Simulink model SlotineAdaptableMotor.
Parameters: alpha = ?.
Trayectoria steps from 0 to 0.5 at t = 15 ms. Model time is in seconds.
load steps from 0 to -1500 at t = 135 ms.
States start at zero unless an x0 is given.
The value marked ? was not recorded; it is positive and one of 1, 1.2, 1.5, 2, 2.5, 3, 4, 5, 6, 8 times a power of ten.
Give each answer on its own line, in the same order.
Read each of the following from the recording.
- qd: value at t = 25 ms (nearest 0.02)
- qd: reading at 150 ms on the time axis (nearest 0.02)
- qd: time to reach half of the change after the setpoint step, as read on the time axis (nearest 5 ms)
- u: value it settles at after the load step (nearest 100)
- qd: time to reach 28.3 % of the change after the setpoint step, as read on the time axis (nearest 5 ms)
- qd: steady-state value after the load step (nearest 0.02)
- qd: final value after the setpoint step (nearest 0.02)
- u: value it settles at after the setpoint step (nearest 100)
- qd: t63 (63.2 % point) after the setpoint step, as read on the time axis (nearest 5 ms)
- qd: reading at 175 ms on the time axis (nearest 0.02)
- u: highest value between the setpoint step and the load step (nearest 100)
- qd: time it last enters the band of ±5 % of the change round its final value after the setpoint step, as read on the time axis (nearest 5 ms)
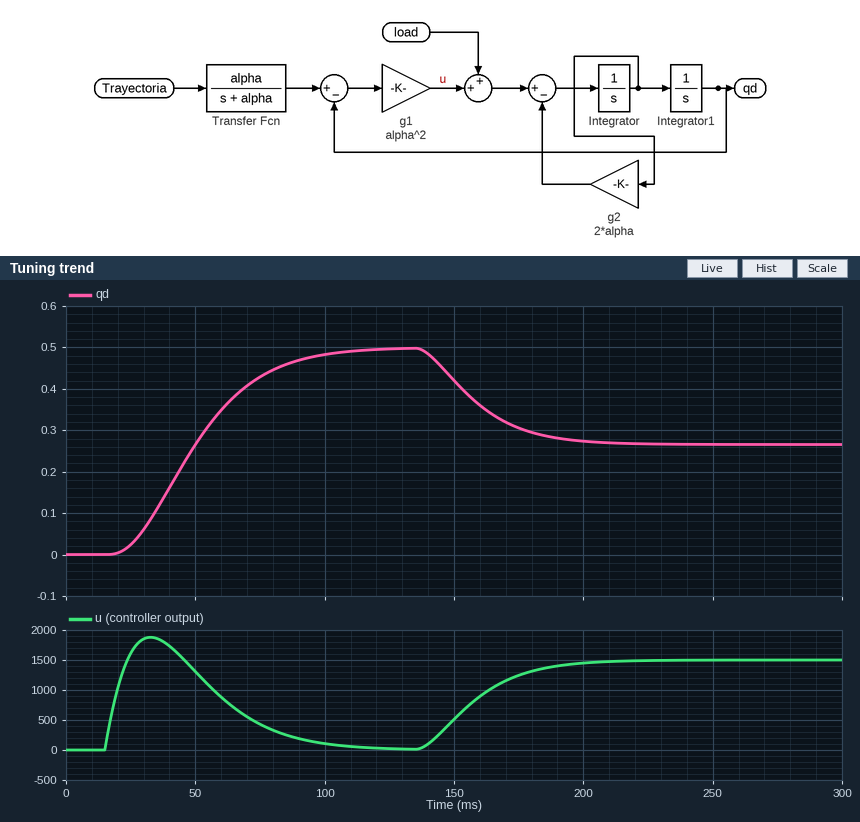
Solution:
0.02
0.42
50 ms
1500
40 ms
0.26
0.50
0
55 ms
0.30
1900
95 ms
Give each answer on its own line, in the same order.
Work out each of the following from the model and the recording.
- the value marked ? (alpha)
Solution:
80
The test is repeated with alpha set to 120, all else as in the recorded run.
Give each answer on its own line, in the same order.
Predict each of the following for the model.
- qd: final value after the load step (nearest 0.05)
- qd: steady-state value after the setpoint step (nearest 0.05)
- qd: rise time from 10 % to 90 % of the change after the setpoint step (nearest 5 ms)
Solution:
0.40
0.50
35 ms
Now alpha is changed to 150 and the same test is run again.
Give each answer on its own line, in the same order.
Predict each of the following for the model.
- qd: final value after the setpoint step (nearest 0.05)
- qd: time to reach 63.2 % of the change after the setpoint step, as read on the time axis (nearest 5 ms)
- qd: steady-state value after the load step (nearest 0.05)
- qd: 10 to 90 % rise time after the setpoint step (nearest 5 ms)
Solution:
0.50
35 ms
0.45
30 ms
